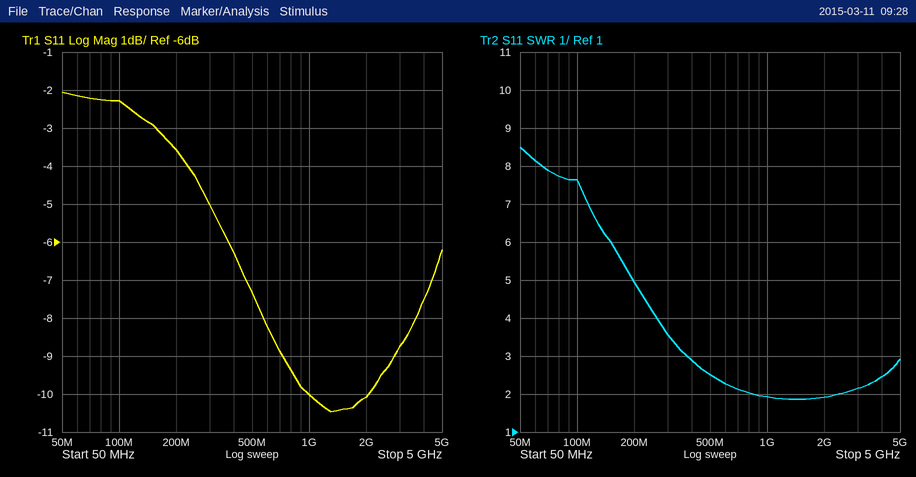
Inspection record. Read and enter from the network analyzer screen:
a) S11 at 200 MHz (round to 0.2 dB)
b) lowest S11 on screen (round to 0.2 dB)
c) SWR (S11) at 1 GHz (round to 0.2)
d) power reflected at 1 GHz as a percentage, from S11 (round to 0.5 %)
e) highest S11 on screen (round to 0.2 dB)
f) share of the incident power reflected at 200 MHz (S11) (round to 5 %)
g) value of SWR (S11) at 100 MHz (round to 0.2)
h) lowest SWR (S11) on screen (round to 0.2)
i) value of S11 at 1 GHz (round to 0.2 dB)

-3.6 dB
-10.4 dB
2.0
10.0 %
-2.0 dB
45 %
7.6
1.8
-10.0 dB
